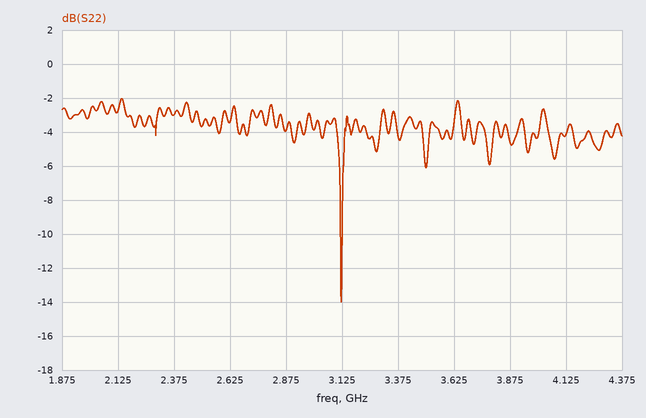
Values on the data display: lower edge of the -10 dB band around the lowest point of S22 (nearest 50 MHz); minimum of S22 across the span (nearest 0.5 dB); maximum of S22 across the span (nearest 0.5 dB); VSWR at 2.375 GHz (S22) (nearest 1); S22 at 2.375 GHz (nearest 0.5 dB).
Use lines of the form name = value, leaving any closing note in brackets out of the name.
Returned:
lower edge of the -10 dB band around the lowest point of S22 = 3.10 GHz
minimum of S22 across the span = -14.0 dB
maximum of S22 across the span = -2.0 dB
VSWR at 2.375 GHz (S22) = 6
S22 at 2.375 GHz = -3.0 dB
